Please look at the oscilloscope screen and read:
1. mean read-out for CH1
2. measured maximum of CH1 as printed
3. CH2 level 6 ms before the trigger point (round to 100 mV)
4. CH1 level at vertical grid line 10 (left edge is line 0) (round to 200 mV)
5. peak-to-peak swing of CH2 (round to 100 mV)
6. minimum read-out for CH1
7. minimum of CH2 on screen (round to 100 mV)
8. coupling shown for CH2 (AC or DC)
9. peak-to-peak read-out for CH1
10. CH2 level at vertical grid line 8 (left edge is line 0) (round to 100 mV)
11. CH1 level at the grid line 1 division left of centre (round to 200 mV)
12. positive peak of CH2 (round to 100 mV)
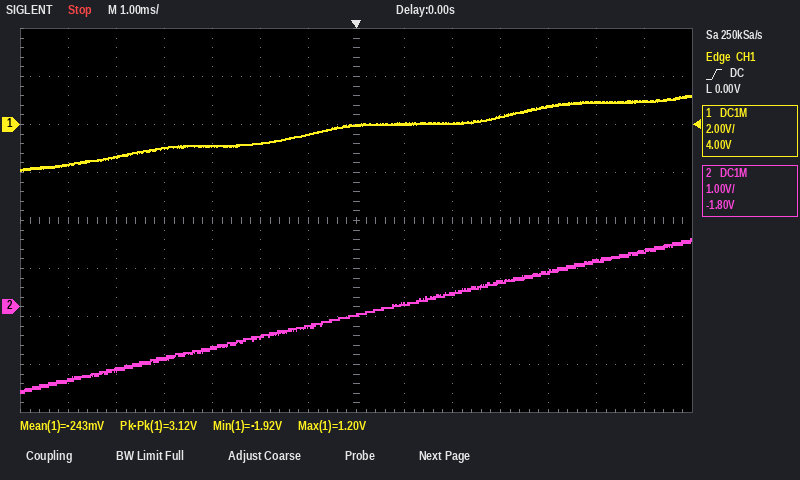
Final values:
-243 mV
1.20 V
-1.5 V
400 mV
3.2 V
-1.92 V
-1.8 V
DC
3.12 V
100 mV
-400 mV
1.4 V
